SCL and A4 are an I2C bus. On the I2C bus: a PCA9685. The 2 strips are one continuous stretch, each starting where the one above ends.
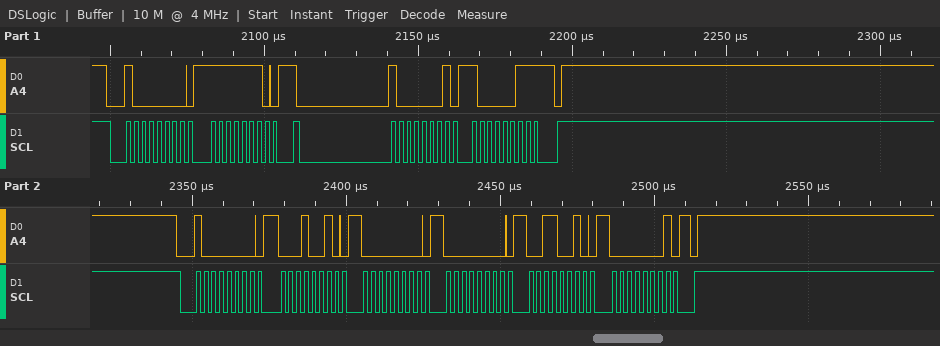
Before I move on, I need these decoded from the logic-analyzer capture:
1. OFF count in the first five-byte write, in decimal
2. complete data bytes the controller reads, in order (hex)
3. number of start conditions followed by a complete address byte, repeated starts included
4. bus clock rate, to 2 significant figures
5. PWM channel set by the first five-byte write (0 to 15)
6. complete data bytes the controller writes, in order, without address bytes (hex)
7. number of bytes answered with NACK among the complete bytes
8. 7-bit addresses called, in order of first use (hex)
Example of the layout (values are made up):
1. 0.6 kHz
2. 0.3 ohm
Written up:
1. 306
2. 83
3. 3
4. 400 kHz
5. 3
6. FE 12 00 00 32 01
7. 1
8. 0x40
